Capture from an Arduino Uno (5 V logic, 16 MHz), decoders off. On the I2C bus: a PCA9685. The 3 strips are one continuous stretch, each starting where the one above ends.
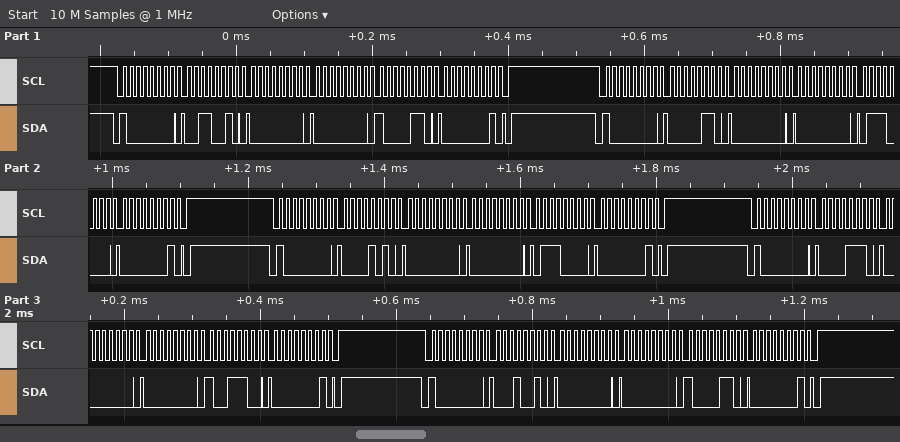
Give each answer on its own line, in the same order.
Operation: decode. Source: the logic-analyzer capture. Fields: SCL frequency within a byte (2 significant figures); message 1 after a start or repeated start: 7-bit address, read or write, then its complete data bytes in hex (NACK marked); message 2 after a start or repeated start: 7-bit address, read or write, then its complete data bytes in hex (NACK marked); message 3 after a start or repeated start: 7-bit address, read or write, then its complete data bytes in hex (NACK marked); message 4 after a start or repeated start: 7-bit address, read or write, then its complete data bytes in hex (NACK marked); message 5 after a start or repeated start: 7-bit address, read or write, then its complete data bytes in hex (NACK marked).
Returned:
100 kHz
0x40 write: 32 00 00 86 01
0x40 write: 06 00 00 70 01
0x40 write: 0A 00 00 70 01
0x40 write: 0E 00 00 9C 01
0x40 write: 12 00 00 86 01
